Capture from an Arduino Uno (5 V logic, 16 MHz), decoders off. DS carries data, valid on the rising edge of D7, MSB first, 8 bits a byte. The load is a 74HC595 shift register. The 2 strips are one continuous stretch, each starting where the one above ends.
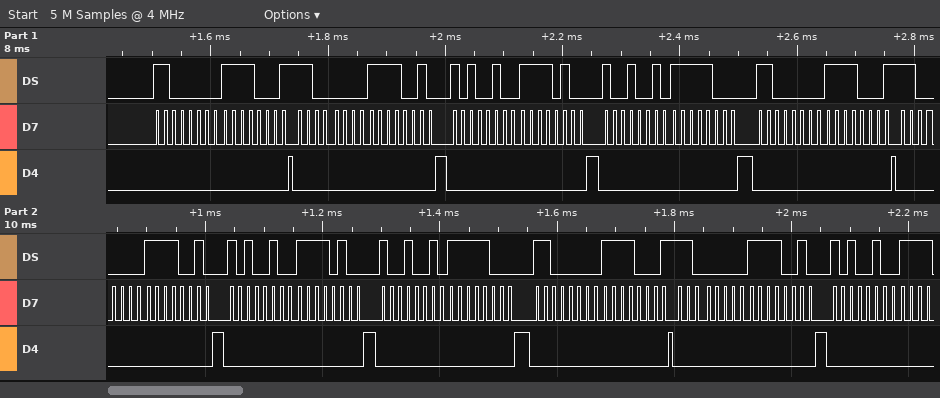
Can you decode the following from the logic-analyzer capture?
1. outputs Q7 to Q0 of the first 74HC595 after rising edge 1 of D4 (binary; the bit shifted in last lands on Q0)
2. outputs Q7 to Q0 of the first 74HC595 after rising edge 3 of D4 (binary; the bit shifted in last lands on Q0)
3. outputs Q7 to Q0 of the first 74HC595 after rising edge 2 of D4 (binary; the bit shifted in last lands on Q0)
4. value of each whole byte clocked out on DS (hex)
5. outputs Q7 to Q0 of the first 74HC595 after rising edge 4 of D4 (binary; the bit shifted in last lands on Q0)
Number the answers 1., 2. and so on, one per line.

1. 11110001
2. 11110100
3. 11110010
4. 0xC0 0xF1 0xC0 0xF2 0xA4 0xF4 0x92 0xF8 0xC0 0xF1 0xC0 0xF2 0xA4 0xF4 0x92 0xF8 0xC0 0xF1 0xC0 0xF2 0xA4
5. 11111000
